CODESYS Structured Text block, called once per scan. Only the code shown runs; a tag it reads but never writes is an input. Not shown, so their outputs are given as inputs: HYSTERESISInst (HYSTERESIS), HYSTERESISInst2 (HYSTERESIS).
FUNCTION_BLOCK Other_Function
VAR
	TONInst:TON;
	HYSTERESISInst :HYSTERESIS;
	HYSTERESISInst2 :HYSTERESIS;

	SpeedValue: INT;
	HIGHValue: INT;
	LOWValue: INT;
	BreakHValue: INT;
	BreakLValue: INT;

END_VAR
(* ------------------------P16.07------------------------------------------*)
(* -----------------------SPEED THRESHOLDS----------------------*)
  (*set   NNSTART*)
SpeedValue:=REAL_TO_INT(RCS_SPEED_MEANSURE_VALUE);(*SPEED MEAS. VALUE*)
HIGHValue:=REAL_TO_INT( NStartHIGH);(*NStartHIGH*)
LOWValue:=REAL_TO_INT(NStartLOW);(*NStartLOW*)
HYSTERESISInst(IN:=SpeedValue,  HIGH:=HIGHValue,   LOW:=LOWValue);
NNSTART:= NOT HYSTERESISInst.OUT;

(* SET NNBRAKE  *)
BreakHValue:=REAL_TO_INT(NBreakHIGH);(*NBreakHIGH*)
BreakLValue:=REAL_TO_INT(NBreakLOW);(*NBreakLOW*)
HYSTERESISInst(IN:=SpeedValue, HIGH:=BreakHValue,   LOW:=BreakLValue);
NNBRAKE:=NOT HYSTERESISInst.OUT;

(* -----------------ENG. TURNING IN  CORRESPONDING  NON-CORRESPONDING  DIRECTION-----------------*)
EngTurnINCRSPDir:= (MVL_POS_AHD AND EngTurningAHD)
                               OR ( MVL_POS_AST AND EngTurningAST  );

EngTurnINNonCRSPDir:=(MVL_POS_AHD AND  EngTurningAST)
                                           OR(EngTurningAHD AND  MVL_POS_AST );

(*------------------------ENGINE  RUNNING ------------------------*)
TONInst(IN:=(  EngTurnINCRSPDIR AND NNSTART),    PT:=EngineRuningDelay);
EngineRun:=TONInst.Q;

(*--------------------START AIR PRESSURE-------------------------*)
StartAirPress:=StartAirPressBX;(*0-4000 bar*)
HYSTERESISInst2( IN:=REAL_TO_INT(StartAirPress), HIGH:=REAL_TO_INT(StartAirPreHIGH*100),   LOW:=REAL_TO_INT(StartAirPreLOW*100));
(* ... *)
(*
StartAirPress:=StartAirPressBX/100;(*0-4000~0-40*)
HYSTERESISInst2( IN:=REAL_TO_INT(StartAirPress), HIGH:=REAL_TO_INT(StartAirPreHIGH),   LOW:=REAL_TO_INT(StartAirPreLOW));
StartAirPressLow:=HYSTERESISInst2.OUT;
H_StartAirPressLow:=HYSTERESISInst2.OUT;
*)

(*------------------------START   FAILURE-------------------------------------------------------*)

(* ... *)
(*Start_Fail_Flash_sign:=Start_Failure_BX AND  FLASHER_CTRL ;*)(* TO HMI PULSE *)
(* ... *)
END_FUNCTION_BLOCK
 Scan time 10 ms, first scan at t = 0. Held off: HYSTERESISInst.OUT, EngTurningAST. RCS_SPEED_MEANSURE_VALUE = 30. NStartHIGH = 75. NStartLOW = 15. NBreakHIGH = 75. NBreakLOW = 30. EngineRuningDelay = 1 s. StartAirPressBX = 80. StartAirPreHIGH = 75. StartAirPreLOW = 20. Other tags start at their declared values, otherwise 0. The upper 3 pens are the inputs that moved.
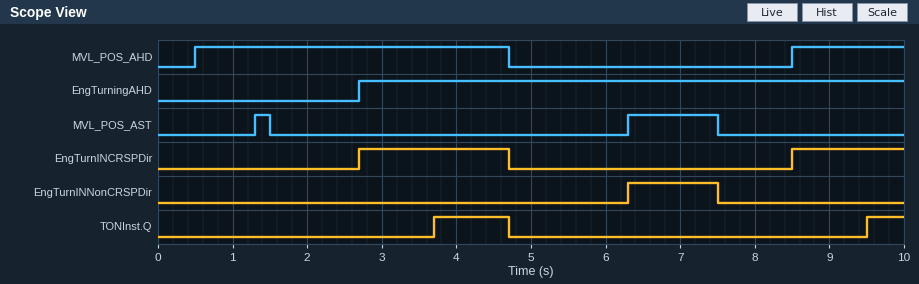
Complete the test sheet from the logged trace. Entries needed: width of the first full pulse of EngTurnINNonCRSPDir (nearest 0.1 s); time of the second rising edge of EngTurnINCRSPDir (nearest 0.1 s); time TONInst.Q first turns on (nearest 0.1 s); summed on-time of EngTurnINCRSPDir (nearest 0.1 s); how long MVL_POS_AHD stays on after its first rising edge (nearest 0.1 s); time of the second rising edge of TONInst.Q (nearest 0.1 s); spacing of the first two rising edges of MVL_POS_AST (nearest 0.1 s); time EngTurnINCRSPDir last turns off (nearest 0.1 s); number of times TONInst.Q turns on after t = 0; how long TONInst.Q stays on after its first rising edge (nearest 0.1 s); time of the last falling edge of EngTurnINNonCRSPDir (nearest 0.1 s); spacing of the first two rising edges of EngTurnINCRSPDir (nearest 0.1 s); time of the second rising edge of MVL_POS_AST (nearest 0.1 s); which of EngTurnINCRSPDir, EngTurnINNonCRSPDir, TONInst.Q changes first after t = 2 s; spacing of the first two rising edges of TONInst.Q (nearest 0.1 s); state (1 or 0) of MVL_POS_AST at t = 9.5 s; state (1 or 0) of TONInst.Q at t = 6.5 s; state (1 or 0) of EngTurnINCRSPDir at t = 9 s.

1.2 s
8.5 s
3.7 s
3.5 s
4.2 s
9.5 s
5.0 s
4.7 s
2
1.0 s
7.5 s
5.8 s
6.3 s
EngTurnINCRSPDir
5.8 s
0
0
1
